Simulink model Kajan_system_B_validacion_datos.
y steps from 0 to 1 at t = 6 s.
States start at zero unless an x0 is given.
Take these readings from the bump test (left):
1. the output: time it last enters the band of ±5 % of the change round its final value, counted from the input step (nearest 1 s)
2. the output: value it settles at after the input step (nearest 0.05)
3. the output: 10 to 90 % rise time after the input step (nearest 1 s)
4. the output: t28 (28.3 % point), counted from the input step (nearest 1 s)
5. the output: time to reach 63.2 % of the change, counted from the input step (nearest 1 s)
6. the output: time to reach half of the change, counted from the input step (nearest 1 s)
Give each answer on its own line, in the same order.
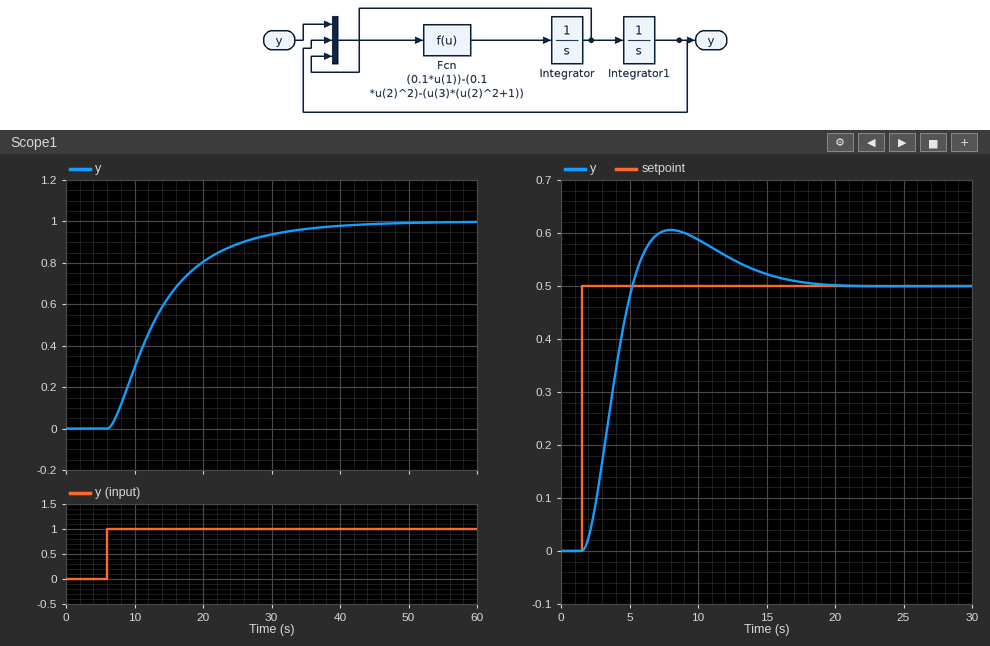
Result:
26 s
1.00
18 s
4 s
9 s
7 s
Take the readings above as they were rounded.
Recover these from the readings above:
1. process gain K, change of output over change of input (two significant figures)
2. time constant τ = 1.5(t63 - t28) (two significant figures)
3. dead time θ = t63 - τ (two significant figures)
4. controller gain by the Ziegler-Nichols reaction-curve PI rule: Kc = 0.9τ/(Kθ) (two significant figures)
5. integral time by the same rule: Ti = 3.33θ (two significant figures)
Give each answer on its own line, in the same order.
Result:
1.0
7.5 s
1.5 s
4.5
5.0 s
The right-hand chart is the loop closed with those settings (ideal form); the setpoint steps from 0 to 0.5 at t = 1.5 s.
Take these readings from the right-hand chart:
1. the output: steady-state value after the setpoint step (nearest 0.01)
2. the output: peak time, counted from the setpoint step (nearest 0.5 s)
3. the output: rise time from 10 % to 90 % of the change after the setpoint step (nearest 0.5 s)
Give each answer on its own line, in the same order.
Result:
0.50
6.5 s
2.5 s
